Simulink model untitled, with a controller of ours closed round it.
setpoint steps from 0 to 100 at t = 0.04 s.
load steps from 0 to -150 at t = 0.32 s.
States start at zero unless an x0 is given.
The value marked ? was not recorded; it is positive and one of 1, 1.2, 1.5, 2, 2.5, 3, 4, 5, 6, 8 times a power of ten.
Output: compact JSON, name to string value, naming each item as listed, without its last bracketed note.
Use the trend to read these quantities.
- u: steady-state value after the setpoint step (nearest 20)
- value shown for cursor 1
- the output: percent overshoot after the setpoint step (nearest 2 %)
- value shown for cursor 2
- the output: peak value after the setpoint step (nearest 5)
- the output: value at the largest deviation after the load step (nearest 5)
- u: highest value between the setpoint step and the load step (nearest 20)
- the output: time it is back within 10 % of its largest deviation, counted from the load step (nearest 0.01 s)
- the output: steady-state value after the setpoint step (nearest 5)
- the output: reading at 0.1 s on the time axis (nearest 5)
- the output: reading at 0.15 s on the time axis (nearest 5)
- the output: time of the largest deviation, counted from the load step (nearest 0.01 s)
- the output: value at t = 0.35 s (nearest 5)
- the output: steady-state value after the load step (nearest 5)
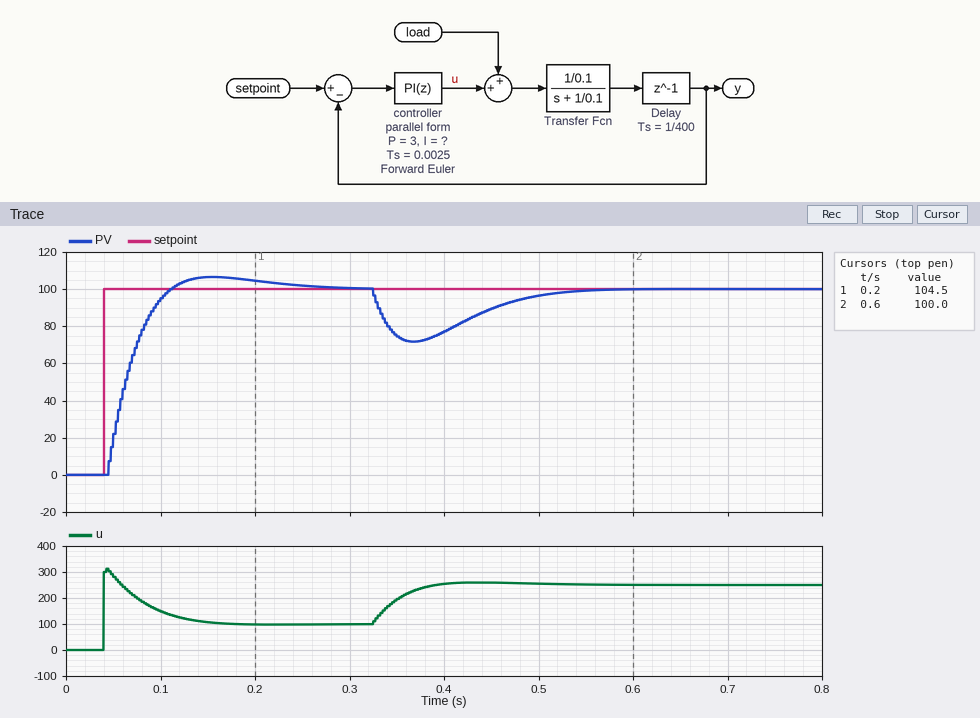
{"u: steady-state value after the setpoint step": "100", "value shown for cursor 1": "104.5", "the output: percent overshoot after the setpoint step": "6 %", "value shown for cursor 2": "100.0", "the output: peak value after the setpoint step": "105", "the output: value at the largest deviation after the load step": "70", "u: highest value between the setpoint step and the load step": "320", "the output: time it is back within 10 % of its largest deviation, counted from the load step": "0.19 s", "the output: steady-state value after the setpoint step": "100", "the output: reading at 0.1 s on the time axis": "95", "the output: reading at 0.15 s on the time axis": "105", "the output: time of the largest deviation, counted from the load step": "0.05 s", "the output: value at t = 0.35 s": "75", "the output: steady-state value after the load step": "100"}
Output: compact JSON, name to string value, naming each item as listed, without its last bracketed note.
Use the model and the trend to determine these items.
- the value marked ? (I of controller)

{"the value marked ?": "50"}
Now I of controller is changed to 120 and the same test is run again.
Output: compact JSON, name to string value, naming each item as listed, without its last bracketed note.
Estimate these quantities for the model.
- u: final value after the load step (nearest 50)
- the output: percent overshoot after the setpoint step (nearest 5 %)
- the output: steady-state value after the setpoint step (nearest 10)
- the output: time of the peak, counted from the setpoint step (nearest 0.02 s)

{"u: final value after the load step": "250", "the output: percent overshoot after the setpoint step": "25 %", "the output: steady-state value after the setpoint step": "100", "the output: time of the peak, counted from the setpoint step": "0.08 s"}
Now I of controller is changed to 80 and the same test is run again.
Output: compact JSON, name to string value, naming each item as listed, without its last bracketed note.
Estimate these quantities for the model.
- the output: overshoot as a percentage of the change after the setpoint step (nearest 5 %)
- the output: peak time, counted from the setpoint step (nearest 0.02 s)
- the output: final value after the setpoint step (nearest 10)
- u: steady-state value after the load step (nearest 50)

{"the output: overshoot as a percentage of the change after the setpoint step": "15 %", "the output: peak time, counted from the setpoint step": "0.08 s", "the output: final value after the setpoint step": "100", "u: steady-state value after the load step": "250"}
